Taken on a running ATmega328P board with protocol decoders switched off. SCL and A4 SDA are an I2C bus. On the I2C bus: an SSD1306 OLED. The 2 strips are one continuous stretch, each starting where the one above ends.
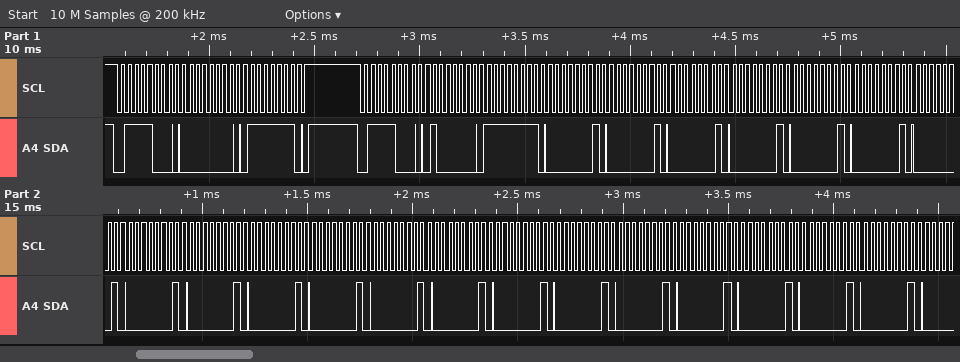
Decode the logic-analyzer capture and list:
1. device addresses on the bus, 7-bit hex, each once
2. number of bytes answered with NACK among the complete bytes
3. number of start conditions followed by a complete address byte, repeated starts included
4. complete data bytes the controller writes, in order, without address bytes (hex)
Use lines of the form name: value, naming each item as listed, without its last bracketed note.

device addresses on the bus, 7-bit hex, each once: 0x3C
number of bytes answered with NACK among the complete bytes: 0
number of start conditions followed by a complete address byte, repeated starts included: 2
complete data bytes the controller writes, in order, without address bytes: 00 7F 40 FF 01 01 01 01 01 01 01 01 01 01 01 01 01 01 01 01 01 01 01 01
